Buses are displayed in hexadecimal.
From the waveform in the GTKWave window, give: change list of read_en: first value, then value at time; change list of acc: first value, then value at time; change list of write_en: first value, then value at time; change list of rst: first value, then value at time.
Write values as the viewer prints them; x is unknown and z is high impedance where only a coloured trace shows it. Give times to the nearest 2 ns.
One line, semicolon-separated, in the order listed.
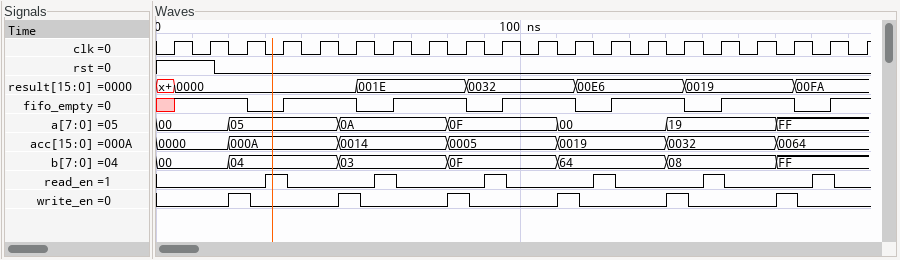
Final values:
0, 1 at 30 ns, 0 at 36 ns, 1 at 60 ns, 0 at 66 ns, 1 at 90 ns, 0 at 96 ns, 1 at 120 ns, 0 at 126 ns, 1 at 150 ns, 0 at 156 ns, 1 at 180 ns, 0 at 186 ns; 0000, 000A at 20 ns, 0014 at 50 ns, 0005 at 80 ns, 0019 at 110 ns, 0032 at 140 ns, 0064 at 170 ns; 0, 1 at 20 ns, 0 at 26 ns, 1 at 50 ns, 0 at 56 ns, 1 at 80 ns, 0 at 86 ns, 1 at 110 ns, 0 at 116 ns, 1 at 140 ns, 0 at 146 ns, 1 at 170 ns, 0 at 176 ns; 1, 0 at 16 ns
